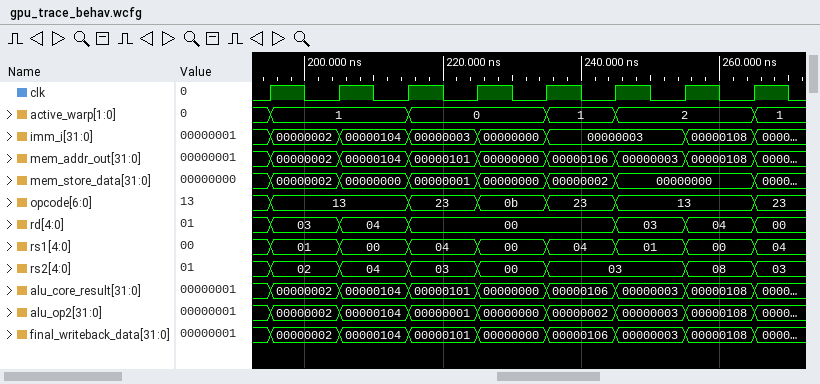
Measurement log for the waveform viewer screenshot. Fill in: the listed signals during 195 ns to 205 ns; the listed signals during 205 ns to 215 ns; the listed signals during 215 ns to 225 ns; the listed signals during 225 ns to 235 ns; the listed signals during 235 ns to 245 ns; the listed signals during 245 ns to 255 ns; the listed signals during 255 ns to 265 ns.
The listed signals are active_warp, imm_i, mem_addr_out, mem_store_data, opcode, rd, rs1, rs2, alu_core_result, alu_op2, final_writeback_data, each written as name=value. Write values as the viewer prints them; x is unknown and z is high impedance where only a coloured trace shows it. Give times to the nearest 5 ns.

active_warp=1, imm_i=00000002, mem_addr_out=00000002, mem_store_data=00000002, opcode=13, rd=03, rs1=01, rs2=02, alu_core_result=00000002, alu_op2=00000002, final_writeback_data=00000002
active_warp=1, imm_i=00000104, mem_addr_out=00000104, mem_store_data=00000000, opcode=13, rd=04, rs1=00, rs2=04, alu_core_result=00000104, alu_op2=00000104, final_writeback_data=00000104
active_warp=0, imm_i=00000003, mem_addr_out=00000101, mem_store_data=00000001, opcode=23, rd=00, rs1=04, rs2=03, alu_core_result=00000101, alu_op2=00000001, final_writeback_data=00000101
active_warp=0, imm_i=00000000, mem_addr_out=00000000, mem_store_data=00000000, opcode=0b, rd=00, rs1=00, rs2=00, alu_core_result=00000000, alu_op2=00000000, final_writeback_data=00000000
active_warp=1, imm_i=00000003, mem_addr_out=00000106, mem_store_data=00000002, opcode=23, rd=00, rs1=04, rs2=03, alu_core_result=00000106, alu_op2=00000002, final_writeback_data=00000106
active_warp=2, imm_i=00000003, mem_addr_out=00000003, mem_store_data=00000000, opcode=13, rd=03, rs1=01, rs2=03, alu_core_result=00000003, alu_op2=00000003, final_writeback_data=00000003
active_warp=2, imm_i=00000108, mem_addr_out=00000108, mem_store_data=00000000, opcode=13, rd=04, rs1=00, rs2=08, alu_core_result=00000108, alu_op2=00000108, final_writeback_data=00000108
